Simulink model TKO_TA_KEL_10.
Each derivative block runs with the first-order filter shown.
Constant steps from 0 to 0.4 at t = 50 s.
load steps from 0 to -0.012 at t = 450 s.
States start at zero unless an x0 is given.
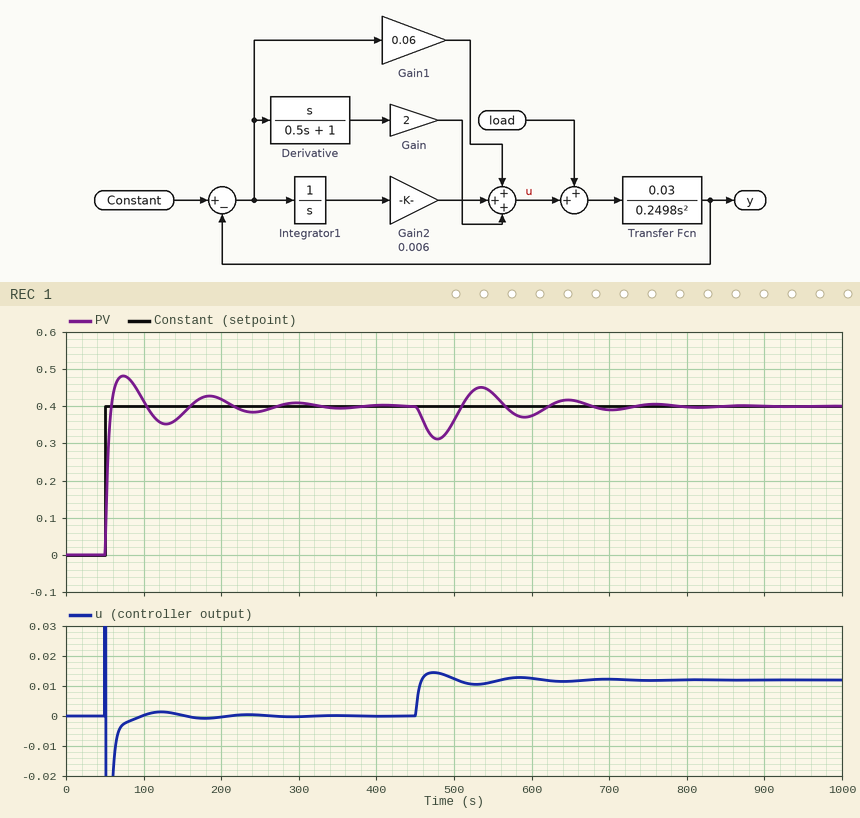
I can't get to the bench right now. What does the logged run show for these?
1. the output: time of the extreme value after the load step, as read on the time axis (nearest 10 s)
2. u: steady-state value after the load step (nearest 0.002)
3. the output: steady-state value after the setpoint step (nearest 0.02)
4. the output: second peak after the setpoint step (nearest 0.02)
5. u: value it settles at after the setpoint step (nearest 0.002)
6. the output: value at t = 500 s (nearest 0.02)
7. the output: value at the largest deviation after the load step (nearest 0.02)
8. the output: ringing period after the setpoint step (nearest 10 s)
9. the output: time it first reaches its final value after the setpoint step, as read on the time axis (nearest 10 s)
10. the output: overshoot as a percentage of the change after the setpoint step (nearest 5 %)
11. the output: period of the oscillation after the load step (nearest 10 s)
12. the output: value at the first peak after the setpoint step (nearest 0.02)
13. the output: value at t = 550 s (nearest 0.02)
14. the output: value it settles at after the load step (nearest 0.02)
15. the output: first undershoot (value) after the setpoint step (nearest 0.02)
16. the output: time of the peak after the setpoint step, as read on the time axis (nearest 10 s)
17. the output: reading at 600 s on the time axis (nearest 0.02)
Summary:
480 s
0.012
0.40
0.42
0.000
0.36
0.32
110 s
60 s
20 %
110 s
0.48
0.44
0.40
0.36
70 s
0.38
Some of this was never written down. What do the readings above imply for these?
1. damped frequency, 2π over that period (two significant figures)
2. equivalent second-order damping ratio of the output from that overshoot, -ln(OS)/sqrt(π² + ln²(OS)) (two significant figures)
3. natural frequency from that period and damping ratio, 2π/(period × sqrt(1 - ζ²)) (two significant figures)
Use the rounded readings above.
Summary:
0.057 rad/s
0.46
0.064 rad/s
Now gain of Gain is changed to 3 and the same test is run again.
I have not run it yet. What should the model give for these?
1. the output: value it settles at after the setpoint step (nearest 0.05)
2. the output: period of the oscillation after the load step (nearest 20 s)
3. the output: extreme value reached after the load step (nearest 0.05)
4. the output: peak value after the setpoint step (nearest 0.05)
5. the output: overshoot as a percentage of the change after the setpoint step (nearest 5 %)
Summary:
0.40
140 s
0.35
0.45
10 %
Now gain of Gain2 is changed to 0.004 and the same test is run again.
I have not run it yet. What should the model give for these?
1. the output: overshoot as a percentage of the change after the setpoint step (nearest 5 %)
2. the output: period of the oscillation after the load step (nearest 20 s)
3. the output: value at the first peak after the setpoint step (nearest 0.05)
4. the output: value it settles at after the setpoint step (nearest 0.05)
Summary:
15 %
140 s
0.45
0.40
